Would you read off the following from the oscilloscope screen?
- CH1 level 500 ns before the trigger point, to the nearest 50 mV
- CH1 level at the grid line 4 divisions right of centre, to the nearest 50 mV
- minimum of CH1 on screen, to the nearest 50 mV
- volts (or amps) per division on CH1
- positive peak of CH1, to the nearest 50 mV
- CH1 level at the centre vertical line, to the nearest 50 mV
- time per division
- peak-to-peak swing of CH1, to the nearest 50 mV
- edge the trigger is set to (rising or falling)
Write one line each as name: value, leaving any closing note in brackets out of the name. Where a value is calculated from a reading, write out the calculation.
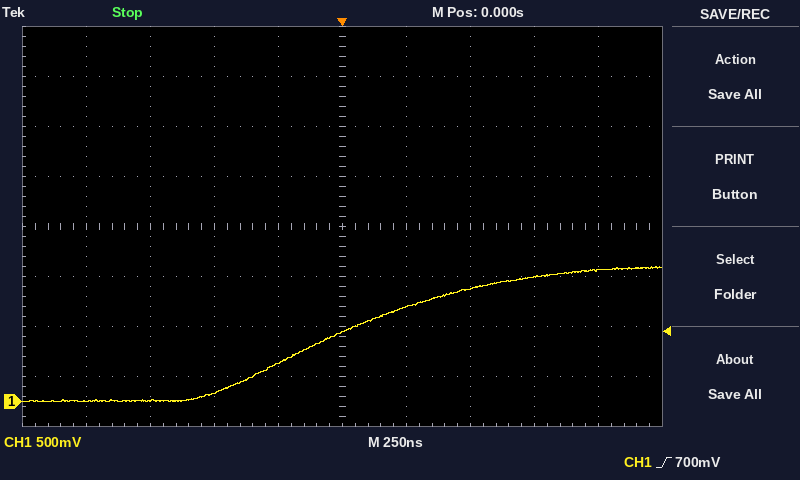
CH1 level 500 ns before the trigger point, to the nearest 50 mV: 100 mV
CH1 level at the grid line 4 divisions right of centre, to the nearest 50 mV: 1.30 V
minimum of CH1 on screen, to the nearest 50 mV: 0 mV
volts (or amps) per division on CH1: 500 mV
positive peak of CH1, to the nearest 50 mV: 1.35 V
CH1 level at the centre vertical line, to the nearest 50 mV: 700 mV
time per division: 250 ns
peak-to-peak swing of CH1, to the nearest 50 mV: 1.35 V − (0 mV) = 1.35 V
edge the trigger is set to: rising
